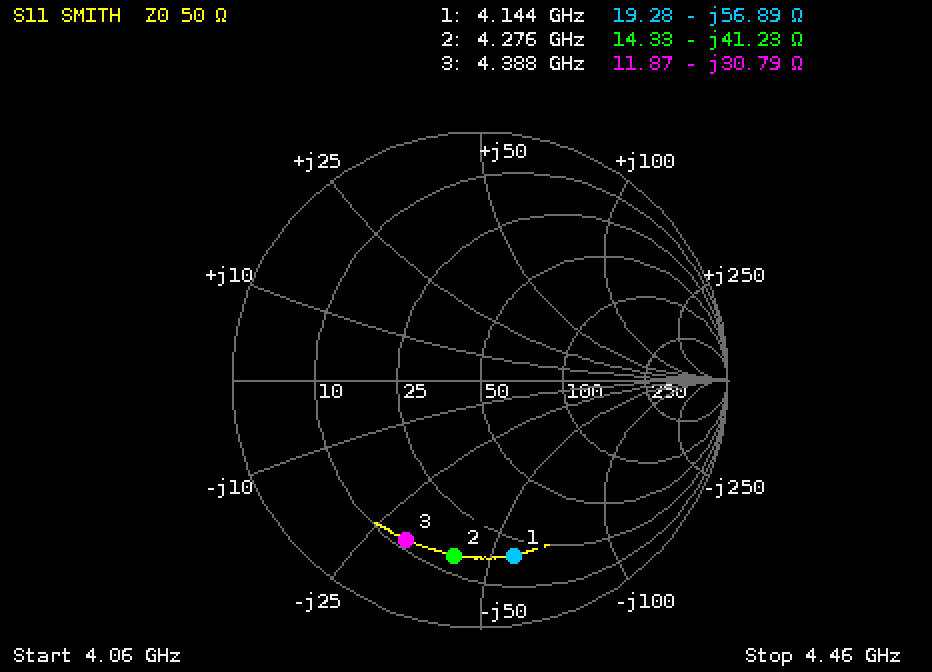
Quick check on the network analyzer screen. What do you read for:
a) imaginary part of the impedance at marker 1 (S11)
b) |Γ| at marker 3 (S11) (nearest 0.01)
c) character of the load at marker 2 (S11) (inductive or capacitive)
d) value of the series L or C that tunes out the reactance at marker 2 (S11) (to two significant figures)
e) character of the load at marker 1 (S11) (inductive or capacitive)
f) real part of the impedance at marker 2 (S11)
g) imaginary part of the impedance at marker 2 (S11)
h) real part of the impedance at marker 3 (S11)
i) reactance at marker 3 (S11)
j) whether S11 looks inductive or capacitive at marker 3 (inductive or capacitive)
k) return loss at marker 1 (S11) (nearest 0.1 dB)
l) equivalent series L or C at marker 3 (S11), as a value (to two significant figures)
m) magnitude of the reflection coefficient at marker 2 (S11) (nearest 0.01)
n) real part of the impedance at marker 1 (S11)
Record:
-56.89 Ω
0.71
capacitive
1.5 nH
capacitive
14.33 Ω
-41.23 Ω
11.87 Ω
-30.79 Ω
capacitive
2.8 dB
1.2 pF
0.71
19.28 Ω
